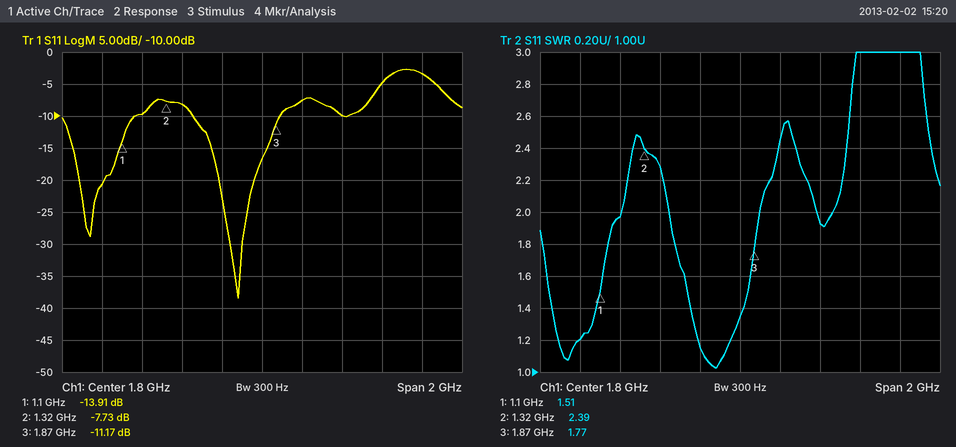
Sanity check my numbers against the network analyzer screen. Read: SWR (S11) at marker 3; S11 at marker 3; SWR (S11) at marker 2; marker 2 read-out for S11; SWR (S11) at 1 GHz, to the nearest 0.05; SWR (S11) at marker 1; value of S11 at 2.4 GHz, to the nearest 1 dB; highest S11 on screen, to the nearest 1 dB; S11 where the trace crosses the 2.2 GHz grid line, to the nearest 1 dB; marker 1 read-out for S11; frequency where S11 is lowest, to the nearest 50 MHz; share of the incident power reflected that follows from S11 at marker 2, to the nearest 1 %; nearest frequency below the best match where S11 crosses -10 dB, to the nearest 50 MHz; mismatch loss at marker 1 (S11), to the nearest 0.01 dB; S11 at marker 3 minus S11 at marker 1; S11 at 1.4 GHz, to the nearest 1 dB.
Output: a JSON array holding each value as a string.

["1.77", "-11.17 dB", "2.39", "-7.73 dB", "1.20", "1.51", "-5 dB", "-3 dB", "-10 dB", "-13.91 dB", "1.70 GHz", "17 %", "1.45 GHz", "0.18 dB", "2.74 dB", "-8 dB"]
